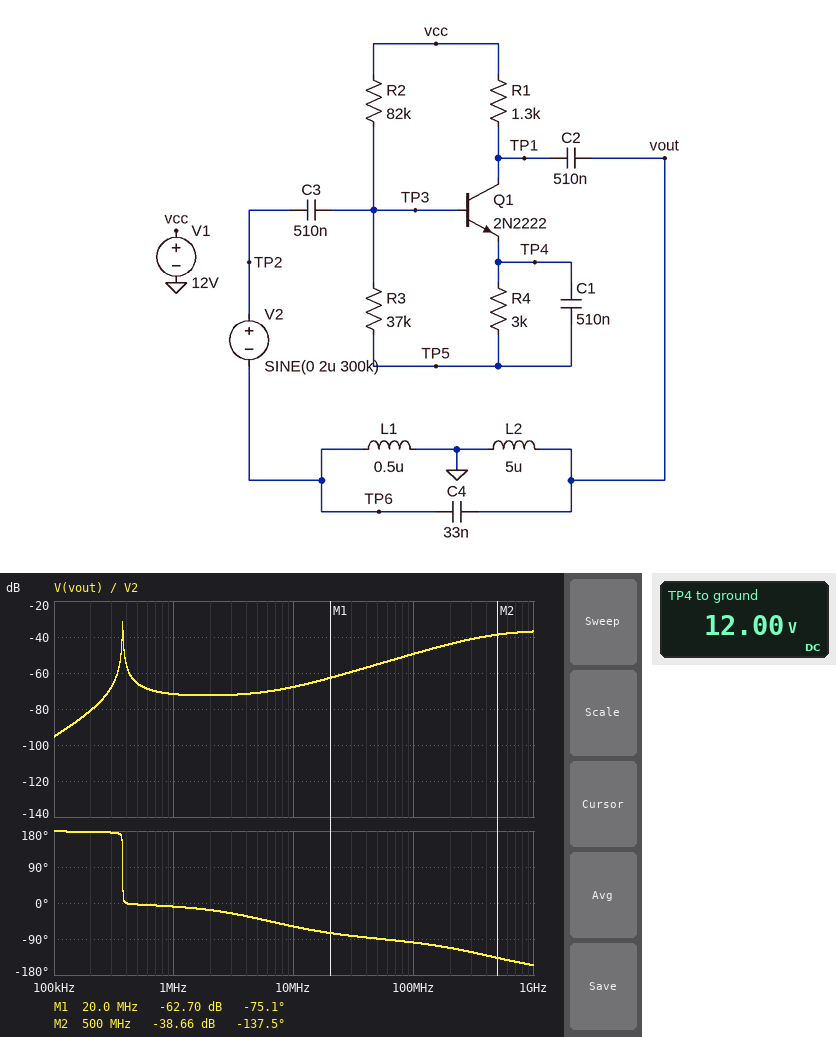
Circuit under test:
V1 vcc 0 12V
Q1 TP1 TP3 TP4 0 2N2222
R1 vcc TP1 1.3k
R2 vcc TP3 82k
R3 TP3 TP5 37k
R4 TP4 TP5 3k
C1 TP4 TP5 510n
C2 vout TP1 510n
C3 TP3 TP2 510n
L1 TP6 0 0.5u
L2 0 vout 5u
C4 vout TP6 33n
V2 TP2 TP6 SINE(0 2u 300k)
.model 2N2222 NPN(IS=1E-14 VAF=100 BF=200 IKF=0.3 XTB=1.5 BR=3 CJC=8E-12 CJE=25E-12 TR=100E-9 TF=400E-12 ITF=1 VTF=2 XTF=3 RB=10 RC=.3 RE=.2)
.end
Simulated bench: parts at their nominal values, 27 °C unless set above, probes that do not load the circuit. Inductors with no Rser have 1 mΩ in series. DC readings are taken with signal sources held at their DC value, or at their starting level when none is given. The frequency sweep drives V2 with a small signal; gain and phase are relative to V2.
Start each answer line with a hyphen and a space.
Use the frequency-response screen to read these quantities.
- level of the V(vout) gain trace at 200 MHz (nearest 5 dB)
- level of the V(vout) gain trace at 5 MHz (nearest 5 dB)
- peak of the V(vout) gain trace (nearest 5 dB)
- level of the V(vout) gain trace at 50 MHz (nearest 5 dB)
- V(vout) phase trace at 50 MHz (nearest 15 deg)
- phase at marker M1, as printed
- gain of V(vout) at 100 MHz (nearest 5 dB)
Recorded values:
- -45 dB
- -70 dB
- -30 dB
- -55 dB
- -90 deg
- -75.1 deg
- -50 dB
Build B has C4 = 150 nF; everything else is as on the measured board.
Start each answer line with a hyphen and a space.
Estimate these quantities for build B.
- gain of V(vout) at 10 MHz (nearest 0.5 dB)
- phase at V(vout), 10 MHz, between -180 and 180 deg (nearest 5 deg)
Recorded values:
- -69.0 dB
- -85 deg
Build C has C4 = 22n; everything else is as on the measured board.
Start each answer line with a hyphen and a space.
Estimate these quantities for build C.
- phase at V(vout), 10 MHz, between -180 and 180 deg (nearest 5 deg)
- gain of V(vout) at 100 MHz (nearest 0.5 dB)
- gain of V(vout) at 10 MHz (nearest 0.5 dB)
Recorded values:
- -50 deg
- -49.5 dB
- -66.5 dB
